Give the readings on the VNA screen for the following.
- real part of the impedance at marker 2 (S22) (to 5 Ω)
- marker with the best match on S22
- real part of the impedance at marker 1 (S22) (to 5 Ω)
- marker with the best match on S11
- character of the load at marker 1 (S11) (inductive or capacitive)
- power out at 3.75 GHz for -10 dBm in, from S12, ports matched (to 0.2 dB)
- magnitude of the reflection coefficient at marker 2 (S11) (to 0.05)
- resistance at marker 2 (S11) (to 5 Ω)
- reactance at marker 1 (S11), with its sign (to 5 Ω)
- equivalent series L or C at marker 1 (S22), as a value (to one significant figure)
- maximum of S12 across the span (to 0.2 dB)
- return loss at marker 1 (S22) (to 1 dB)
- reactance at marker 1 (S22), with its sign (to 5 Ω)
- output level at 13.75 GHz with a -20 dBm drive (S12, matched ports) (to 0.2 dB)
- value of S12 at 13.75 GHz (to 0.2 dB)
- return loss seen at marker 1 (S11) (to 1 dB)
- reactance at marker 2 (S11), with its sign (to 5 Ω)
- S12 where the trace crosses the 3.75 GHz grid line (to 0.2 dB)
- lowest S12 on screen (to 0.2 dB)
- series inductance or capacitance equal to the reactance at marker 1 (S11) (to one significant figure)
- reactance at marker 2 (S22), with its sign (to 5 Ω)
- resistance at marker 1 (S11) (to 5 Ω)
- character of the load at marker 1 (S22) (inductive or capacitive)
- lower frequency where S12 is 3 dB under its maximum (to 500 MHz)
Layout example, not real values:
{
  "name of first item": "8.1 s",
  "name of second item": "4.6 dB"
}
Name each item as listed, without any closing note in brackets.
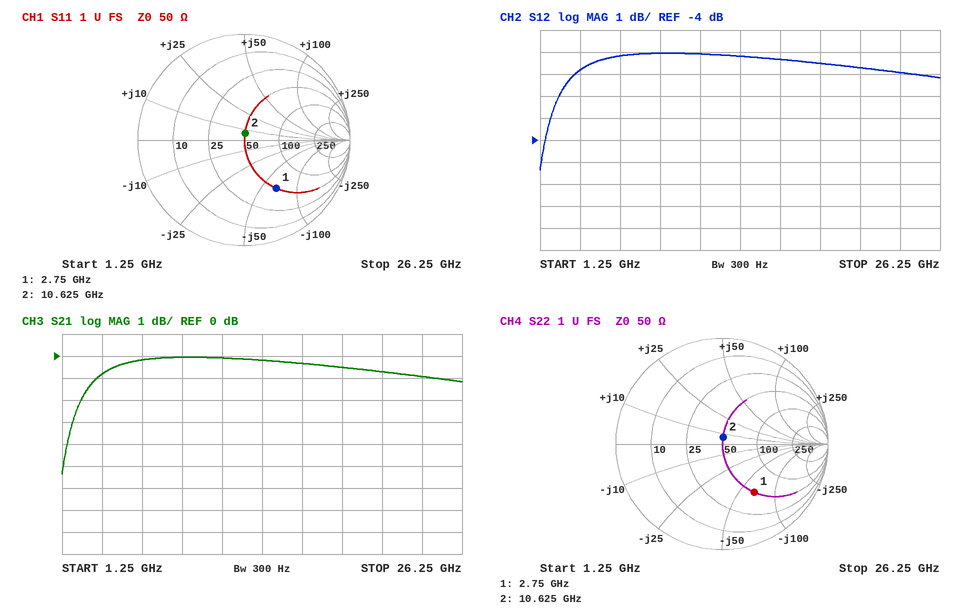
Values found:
{
  "real part of the impedance at marker 2 (S22)": "50 Ω",
  "marker with the best match on S22": "marker 2",
  "real part of the impedance at marker 1 (S22)": "50 Ω",
  "marker with the best match on S11": "marker 2",
  "character of the load at marker 1 (S11)": "capacitive",
  "power out at 3.75 GHz for -10 dBm in, from S12, ports matched": "-10.8 dBm",
  "magnitude of the reflection coefficient at marker 2 (S11)": "0.05",
  "resistance at marker 2 (S11)": "50 Ω",
  "reactance at marker 1 (S11), with its sign": "-65 Ω",
  "equivalent series L or C at marker 1 (S22), as a value": "900 fF",
  "maximum of S12 across the span": "0.0 dB",
  "return loss at marker 1 (S22)": "5 dB",
  "reactance at marker 1 (S22), with its sign": "-65 Ω",
  "output level at 13.75 GHz with a -20 dBm drive (S12, matched ports)": "-20.2 dBm",
  "value of S12 at 13.75 GHz": "-0.2 dB",
  "return loss seen at marker 1 (S11)": "5 dB",
  "reactance at marker 2 (S11), with its sign": "+5 Ω",
  "S12 where the trace crosses the 3.75 GHz grid line": "-0.8 dB",
  "lowest S12 on screen": "-5.4 dB",
  "series inductance or capacitance equal to the reactance at marker 1 (S11)": "900 fF",
  "reactance at marker 2 (S22), with its sign": "+5 Ω",
  "resistance at marker 1 (S11)": "50 Ω",
  "character of the load at marker 1 (S22)": "capacitive",
  "lower frequency where S12 is 3 dB under its maximum": "2.0 GHz"
}
